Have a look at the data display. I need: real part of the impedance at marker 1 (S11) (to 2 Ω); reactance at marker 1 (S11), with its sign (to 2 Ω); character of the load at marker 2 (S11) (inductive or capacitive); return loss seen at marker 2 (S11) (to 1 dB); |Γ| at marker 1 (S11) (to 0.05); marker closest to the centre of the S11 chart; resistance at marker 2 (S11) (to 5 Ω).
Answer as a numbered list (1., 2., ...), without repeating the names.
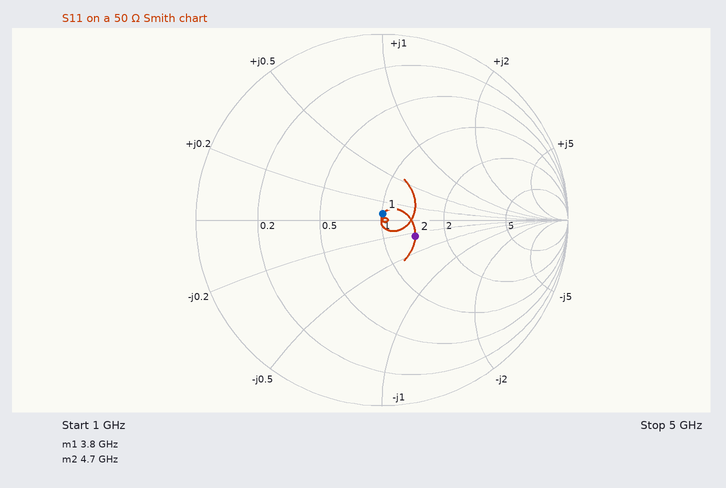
1. 50 Ω
2. +4 Ω
3. capacitive
4. 14 dB
5. 0.05
6. marker 1
7. 70 Ω
